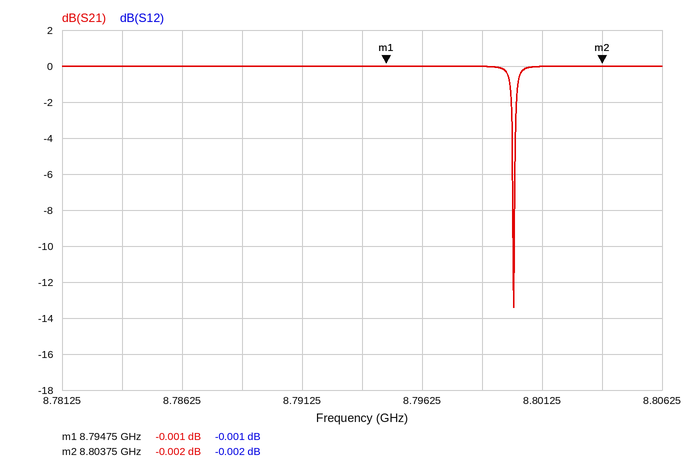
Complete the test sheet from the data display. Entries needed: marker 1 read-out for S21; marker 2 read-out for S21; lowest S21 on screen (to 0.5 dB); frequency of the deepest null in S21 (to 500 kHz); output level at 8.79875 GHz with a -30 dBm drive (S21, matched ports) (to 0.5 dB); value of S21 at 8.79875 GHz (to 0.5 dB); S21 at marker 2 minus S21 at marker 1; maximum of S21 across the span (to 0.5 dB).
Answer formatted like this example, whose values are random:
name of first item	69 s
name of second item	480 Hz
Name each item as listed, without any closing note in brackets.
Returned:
marker 1 read-out for S21	-0.001 dB
marker 2 read-out for S21	-0.002 dB
lowest S21 on screen	-13.5 dB
frequency of the deepest null in S21	8.8000 GHz
output level at 8.79875 GHz with a -30 dBm drive (S21, matched ports)	-30.0 dBm
value of S21 at 8.79875 GHz	0.0 dB
S21 at marker 2 minus S21 at marker 1	-0.001 dB
maximum of S21 across the span	0.0 dB
